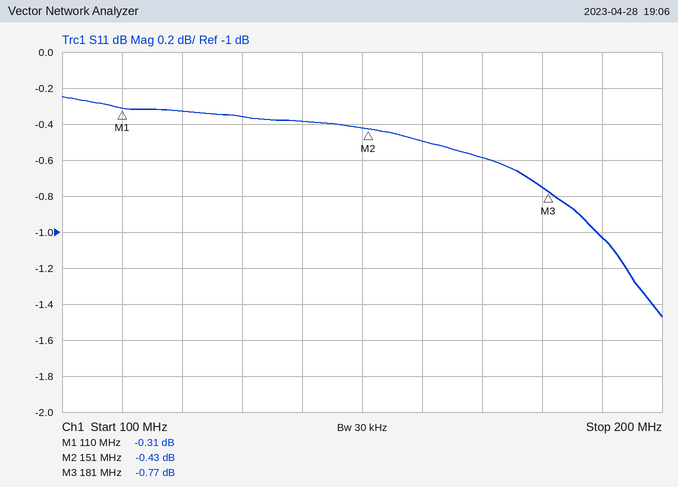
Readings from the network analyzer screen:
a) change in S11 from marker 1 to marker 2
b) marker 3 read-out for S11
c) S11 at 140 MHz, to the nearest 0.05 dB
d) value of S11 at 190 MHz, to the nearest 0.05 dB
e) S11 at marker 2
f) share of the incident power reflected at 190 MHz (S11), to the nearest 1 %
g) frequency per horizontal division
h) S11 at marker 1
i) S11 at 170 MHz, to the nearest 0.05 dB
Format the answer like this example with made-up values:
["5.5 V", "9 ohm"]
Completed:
["-0.12 dB", "-0.77 dB", "-0.40 dB", "-1.05 dB", "-0.43 dB", "79 %", "10 MHz", "-0.31 dB", "-0.60 dB"]
